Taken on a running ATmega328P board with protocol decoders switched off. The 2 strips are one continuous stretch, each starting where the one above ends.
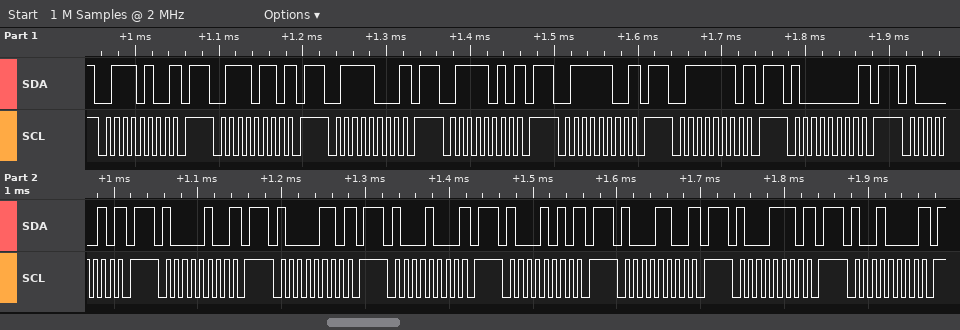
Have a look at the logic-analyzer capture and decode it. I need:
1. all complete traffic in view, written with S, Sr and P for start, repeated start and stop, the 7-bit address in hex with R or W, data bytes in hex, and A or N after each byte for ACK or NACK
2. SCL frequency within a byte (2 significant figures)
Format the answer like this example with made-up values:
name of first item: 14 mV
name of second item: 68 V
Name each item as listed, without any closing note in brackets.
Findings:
all complete traffic in view, written with S, Sr and P for start, repeated start and stop, the 7-bit address in hex with R or W, data bytes in hex, and A or N after each byte for ACK or NACK: S 3AW N P S 3BW N P S 3CW N P S 3DW N P S 3EW N P S 3FW N P S 40W N P S 41W N P S 42W N P S 43W N P S 44W N P S 45W N P S 46W N P S 47W N P S 48W N P
SCL frequency within a byte: 100 kHz
